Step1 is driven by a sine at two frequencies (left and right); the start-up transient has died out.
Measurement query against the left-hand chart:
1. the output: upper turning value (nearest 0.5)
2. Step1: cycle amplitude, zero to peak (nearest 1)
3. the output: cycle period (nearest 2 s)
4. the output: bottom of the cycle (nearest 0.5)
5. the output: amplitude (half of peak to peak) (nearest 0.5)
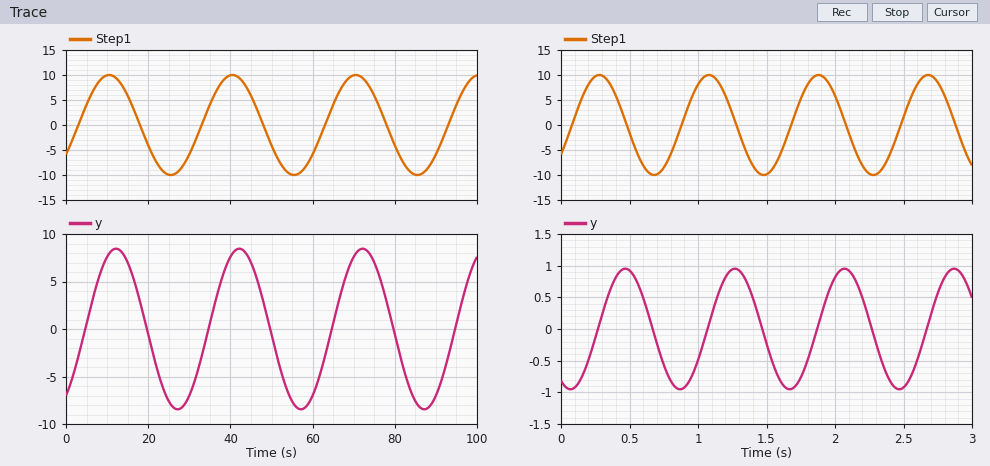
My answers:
8.5
10
30 s
-8.5
8.5
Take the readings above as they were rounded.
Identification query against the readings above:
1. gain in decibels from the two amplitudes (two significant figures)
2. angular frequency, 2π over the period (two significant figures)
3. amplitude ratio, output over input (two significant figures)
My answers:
-1.4 dB
0.21 rad/s
0.85
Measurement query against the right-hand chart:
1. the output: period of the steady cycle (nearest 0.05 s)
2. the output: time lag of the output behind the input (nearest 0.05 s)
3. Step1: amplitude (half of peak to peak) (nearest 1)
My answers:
0.80 s
0.20 s
10
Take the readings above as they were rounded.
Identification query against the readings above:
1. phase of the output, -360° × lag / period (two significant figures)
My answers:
-90°
